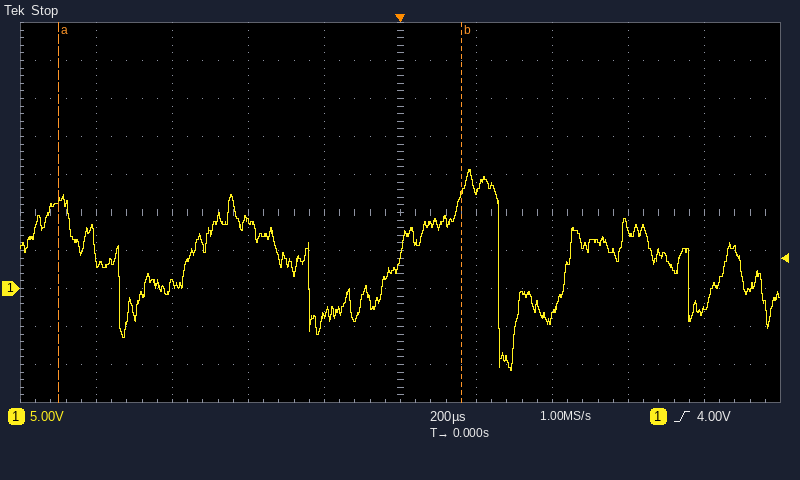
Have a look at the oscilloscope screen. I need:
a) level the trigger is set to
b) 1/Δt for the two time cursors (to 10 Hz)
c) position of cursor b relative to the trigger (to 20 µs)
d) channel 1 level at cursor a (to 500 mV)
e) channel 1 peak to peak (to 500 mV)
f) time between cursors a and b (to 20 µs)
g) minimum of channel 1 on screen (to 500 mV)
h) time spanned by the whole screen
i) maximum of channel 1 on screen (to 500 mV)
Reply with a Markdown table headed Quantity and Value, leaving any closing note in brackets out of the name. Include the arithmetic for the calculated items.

| Quantity | Value |
|---|---|
| level the trigger is set to | 4.00 V |
| 1/Δt for the two time cursors | 1 / 1.06 ms ≈ 940 Hz |
| position of cursor b relative to the trigger | +160 µs |
| channel 1 level at cursor a | 11.5 V |
| channel 1 peak to peak | 15.5 V − (-11.0 V) = 26.5 V |
| time between cursors a and b | 1.06 ms |
| minimum of channel 1 on screen | -11.0 V |
| time spanned by the whole screen | 2 ms |
| maximum of channel 1 on screen | 15.5 V |
